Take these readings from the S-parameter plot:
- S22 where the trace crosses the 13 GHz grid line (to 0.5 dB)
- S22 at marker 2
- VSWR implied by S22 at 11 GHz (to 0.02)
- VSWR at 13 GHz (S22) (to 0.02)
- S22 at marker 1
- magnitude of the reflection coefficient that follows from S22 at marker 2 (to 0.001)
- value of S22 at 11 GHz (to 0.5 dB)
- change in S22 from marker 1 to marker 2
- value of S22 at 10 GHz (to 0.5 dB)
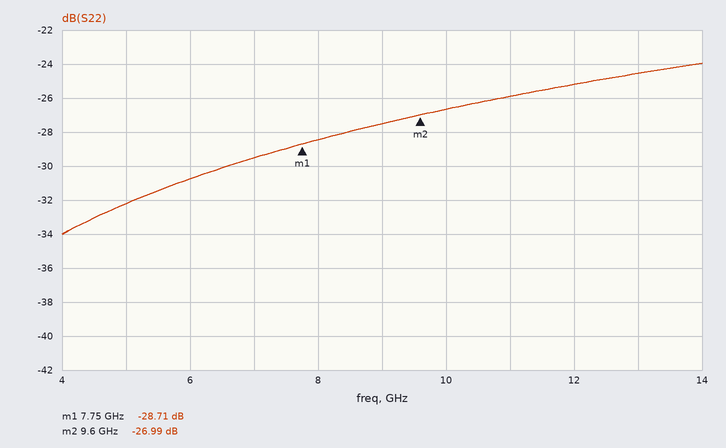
-24.5 dB
-26.99 dB
1.10
1.12
-28.71 dB
0.045
-26.0 dB
1.72 dB
-26.5 dB
